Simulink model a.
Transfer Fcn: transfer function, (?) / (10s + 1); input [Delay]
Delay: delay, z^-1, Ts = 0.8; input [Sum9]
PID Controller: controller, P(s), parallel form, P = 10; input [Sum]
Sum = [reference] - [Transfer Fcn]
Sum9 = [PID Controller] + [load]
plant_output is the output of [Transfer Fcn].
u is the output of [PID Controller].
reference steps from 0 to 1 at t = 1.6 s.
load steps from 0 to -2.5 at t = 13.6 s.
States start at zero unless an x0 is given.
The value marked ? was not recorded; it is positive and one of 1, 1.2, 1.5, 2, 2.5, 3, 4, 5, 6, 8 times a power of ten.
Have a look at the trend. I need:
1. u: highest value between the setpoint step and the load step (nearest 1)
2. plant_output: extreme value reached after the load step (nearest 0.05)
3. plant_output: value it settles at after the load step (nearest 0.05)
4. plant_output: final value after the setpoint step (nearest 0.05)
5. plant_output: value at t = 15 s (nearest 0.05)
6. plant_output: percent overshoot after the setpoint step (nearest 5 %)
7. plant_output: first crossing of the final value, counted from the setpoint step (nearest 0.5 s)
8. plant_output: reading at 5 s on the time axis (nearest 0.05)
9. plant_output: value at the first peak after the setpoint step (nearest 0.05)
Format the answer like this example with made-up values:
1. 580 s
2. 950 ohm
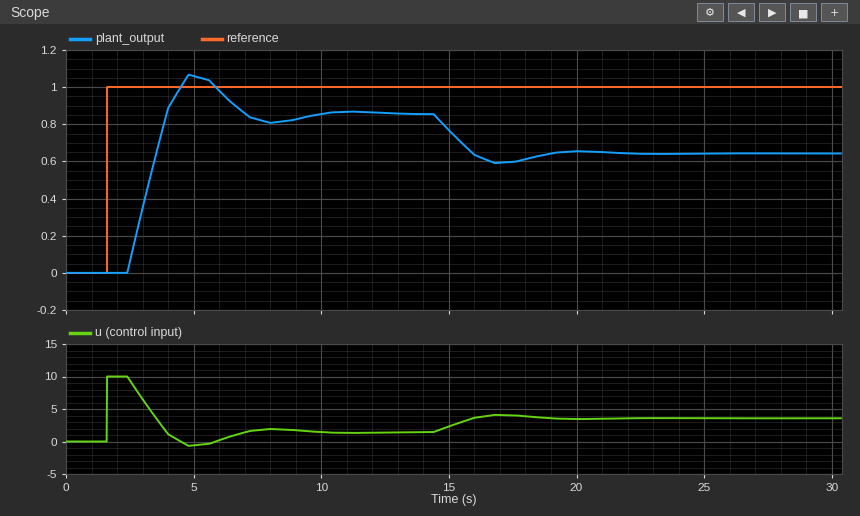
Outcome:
1. 10
2. 0.60
3. 0.65
4. 0.85
5. 0.75
6. 25 %
7. 2.5 s
8. 1.05
9. 1.05
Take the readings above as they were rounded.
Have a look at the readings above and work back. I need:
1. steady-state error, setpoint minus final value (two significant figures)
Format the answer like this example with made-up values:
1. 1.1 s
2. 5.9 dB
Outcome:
1. 0.15
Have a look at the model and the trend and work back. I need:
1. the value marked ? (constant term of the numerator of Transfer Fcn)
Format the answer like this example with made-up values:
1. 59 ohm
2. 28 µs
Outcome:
1. 0.6
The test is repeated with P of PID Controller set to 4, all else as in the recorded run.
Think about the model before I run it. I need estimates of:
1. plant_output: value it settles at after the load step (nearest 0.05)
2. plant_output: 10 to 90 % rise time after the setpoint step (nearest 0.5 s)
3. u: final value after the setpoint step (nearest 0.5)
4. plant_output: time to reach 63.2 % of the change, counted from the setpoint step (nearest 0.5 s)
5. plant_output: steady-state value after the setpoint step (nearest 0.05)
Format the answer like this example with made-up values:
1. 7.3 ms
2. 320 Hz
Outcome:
1. 0.25
2. 4.0 s
3. 1.0
4. 3.0 s
5. 0.70
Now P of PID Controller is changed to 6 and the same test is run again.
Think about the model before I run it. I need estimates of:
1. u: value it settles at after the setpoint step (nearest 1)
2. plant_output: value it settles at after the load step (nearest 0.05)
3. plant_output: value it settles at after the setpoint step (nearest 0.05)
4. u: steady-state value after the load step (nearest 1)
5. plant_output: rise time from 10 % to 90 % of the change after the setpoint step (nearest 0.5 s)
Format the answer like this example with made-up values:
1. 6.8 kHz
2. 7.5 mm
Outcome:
1. 1
2. 0.45
3. 0.80
4. 3
5. 2.5 s
